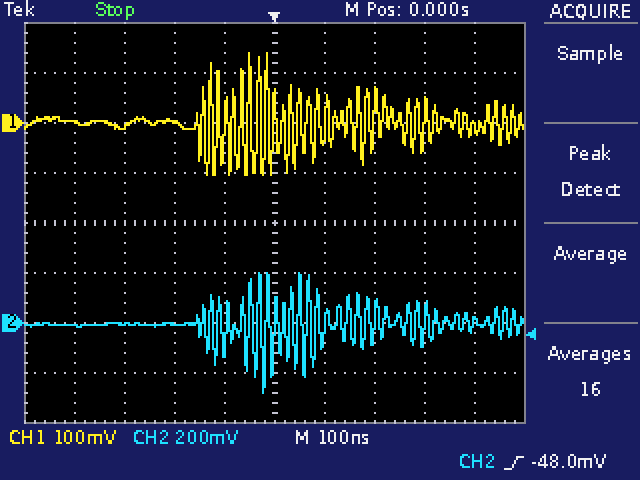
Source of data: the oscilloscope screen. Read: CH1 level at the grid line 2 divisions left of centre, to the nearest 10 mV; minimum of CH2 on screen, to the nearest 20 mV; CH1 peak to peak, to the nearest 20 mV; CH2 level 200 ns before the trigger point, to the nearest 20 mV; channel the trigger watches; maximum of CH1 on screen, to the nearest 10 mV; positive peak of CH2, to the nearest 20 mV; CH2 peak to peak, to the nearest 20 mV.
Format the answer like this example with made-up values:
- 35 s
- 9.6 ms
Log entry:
- 0 mV
- -280 mV
- 240 mV
- 0 mV
- CH2
- 140 mV
- 200 mV
- 480 mV
